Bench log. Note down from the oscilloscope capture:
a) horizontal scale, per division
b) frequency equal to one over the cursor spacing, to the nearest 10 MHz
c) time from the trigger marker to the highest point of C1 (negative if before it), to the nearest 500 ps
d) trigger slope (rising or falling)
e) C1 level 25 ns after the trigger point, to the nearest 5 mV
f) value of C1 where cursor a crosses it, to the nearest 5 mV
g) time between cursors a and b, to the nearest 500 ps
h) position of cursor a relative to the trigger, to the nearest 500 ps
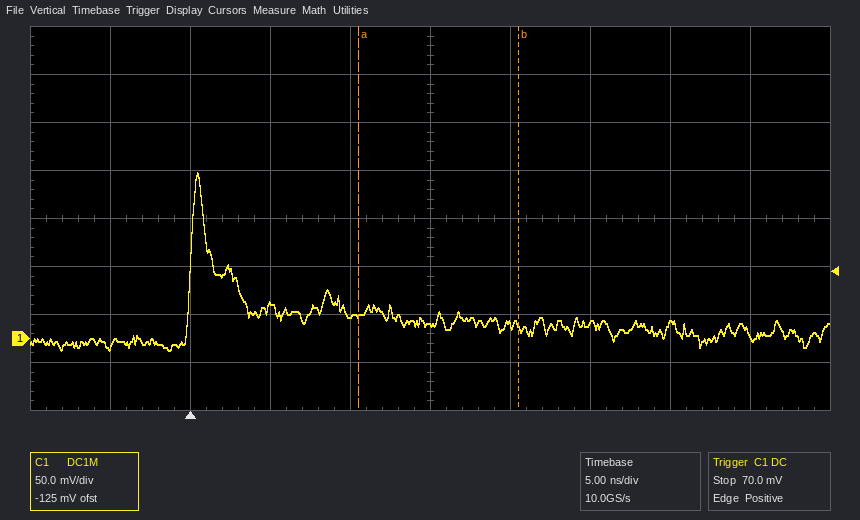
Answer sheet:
5 ns
100 MHz
+500 ps
rising
15 mV
25 mV
10.0 ns
+10.5 ns
